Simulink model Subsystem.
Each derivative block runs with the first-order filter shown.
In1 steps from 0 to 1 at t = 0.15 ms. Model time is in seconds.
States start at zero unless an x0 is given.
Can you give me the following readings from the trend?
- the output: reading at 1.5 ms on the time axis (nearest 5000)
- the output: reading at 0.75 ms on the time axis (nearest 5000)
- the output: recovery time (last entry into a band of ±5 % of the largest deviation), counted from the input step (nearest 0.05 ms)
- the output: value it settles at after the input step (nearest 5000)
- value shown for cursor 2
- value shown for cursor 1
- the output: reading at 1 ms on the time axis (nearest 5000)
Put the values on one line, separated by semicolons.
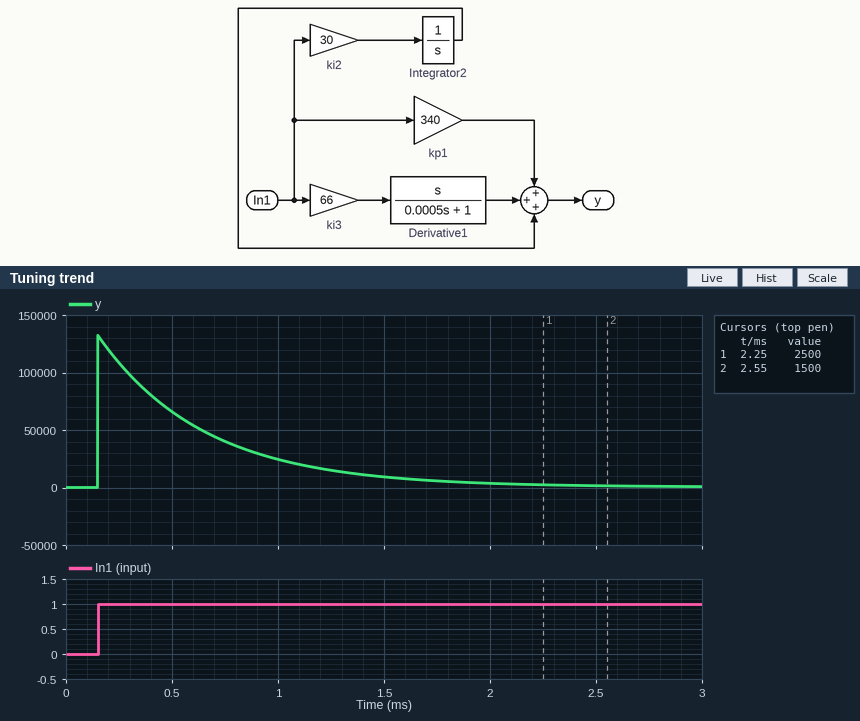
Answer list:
10000; 40000; 1.50 ms; 0; 1500; 2500; 25000
